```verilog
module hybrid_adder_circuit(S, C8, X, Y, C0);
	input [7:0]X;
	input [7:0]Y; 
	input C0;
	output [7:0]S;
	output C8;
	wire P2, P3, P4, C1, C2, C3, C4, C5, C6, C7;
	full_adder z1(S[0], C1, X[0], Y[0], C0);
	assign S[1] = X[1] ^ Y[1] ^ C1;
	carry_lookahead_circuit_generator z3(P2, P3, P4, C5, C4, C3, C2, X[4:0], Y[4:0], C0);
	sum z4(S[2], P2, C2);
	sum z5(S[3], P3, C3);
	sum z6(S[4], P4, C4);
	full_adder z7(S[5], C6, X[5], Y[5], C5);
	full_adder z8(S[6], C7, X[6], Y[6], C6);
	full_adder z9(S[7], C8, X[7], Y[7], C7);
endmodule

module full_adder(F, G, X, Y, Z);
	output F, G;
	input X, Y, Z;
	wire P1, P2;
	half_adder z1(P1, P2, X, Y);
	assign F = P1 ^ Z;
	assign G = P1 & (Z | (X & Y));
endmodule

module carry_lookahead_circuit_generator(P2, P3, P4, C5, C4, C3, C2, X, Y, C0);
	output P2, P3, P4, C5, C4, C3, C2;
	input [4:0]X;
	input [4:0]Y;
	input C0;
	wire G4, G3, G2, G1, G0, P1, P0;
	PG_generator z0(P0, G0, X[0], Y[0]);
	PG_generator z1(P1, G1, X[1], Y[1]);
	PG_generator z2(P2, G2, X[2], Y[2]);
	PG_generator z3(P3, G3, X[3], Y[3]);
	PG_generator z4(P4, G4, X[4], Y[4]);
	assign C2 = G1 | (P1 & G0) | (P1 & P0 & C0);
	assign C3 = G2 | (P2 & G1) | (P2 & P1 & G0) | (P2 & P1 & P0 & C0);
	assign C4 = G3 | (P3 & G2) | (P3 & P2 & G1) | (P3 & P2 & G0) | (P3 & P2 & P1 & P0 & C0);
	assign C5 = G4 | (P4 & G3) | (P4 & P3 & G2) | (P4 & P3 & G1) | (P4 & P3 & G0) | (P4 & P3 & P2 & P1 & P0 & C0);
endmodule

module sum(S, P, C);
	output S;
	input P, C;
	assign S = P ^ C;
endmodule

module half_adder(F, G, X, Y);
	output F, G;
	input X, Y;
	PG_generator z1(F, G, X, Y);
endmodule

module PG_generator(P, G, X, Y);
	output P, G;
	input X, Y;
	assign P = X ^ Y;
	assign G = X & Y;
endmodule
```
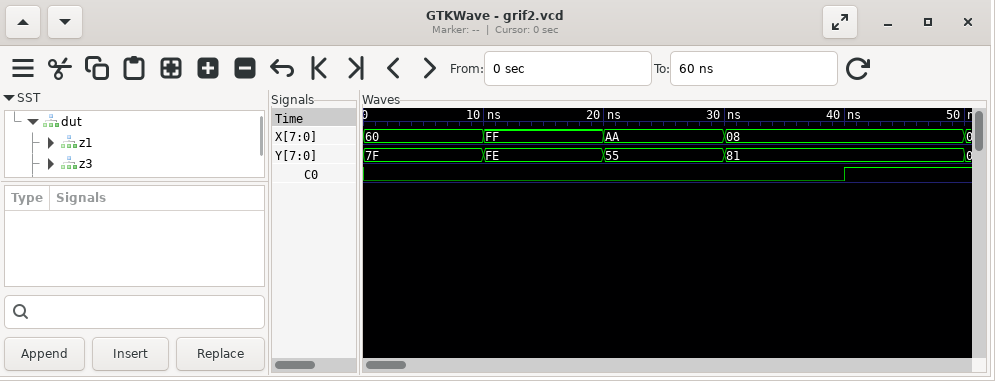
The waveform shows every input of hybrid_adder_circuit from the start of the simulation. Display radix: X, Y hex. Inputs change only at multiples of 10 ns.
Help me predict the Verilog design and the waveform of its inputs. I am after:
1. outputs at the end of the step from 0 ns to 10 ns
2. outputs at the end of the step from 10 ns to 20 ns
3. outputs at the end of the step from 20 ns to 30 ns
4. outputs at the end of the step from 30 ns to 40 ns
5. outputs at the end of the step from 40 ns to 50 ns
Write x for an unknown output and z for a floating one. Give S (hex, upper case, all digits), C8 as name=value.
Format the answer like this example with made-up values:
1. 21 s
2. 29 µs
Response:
1. S=1F, C8=0
2. S=3D, C8=0
3. S=FF, C8=0
4. S=89, C8=0
5. S=8A, C8=0
